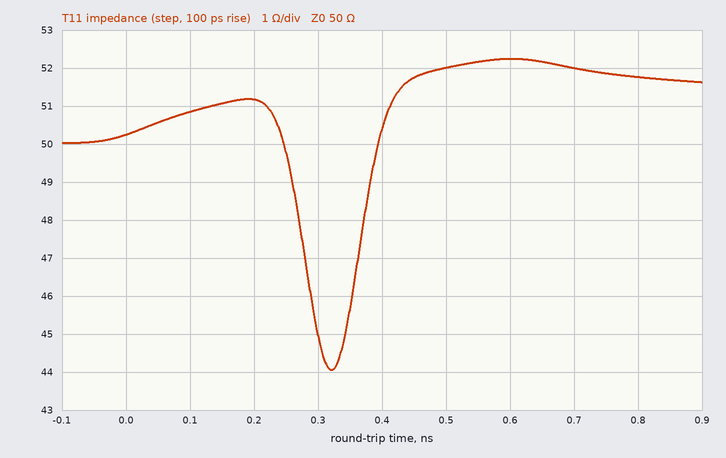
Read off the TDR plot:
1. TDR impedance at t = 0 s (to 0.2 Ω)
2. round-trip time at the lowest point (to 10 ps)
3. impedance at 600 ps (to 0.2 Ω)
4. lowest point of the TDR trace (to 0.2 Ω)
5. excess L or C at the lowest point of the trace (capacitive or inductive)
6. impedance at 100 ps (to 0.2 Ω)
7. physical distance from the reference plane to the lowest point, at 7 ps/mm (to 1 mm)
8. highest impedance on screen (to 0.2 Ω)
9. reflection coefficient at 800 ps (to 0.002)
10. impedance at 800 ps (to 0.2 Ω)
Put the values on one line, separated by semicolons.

50.2 Ω; 320 ps; 52.2 Ω; 44.0 Ω; capacitive; 50.8 Ω; 23 mm; 52.2 Ω; +0.018; 51.8 Ω
